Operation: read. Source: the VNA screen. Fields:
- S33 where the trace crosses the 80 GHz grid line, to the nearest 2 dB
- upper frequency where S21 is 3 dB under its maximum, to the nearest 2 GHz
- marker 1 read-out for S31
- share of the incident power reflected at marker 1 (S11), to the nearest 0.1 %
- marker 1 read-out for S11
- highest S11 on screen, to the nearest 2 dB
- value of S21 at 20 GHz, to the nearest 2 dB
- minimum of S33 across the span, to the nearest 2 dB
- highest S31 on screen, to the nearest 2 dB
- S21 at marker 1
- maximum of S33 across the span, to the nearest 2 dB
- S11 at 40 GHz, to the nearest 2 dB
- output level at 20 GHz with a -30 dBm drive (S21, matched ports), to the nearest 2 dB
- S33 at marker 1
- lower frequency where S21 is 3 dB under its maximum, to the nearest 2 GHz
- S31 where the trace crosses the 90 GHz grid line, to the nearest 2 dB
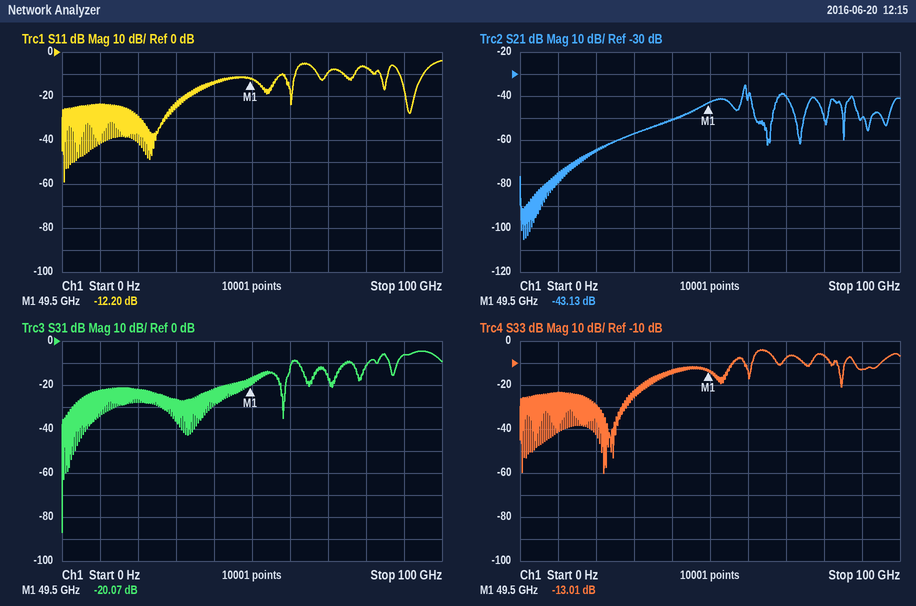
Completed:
-6 dB
60 GHz
-20.07 dB
6.0 %
-12.20 dB
-4 dB
-64 dB
-60 dB
-4 dB
-43.13 dB
-4 dB
-14 dB
-94 dBm
-13.01 dB
58 GHz
-6 dB
